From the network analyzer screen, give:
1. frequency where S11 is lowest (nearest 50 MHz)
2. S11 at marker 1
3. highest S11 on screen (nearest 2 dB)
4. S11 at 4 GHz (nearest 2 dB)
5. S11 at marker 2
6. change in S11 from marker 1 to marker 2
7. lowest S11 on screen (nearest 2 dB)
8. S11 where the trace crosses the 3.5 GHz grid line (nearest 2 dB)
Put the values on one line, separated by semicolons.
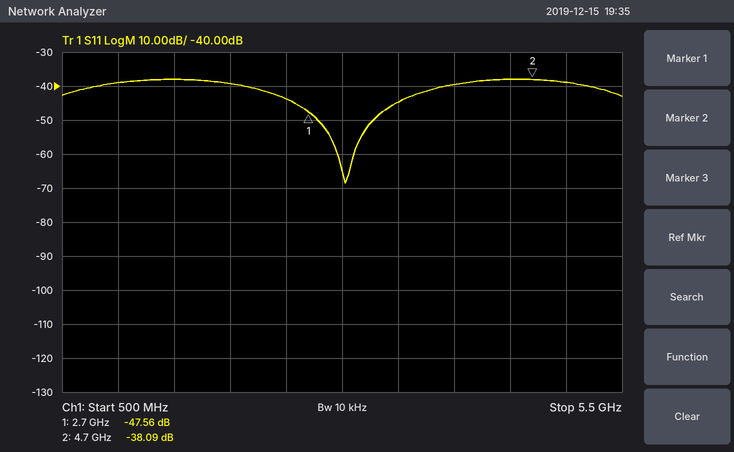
3.05 GHz; -47.56 dB; -38 dB; -40 dB; -38.09 dB; 9.47 dB; -68 dB; -44 dB
